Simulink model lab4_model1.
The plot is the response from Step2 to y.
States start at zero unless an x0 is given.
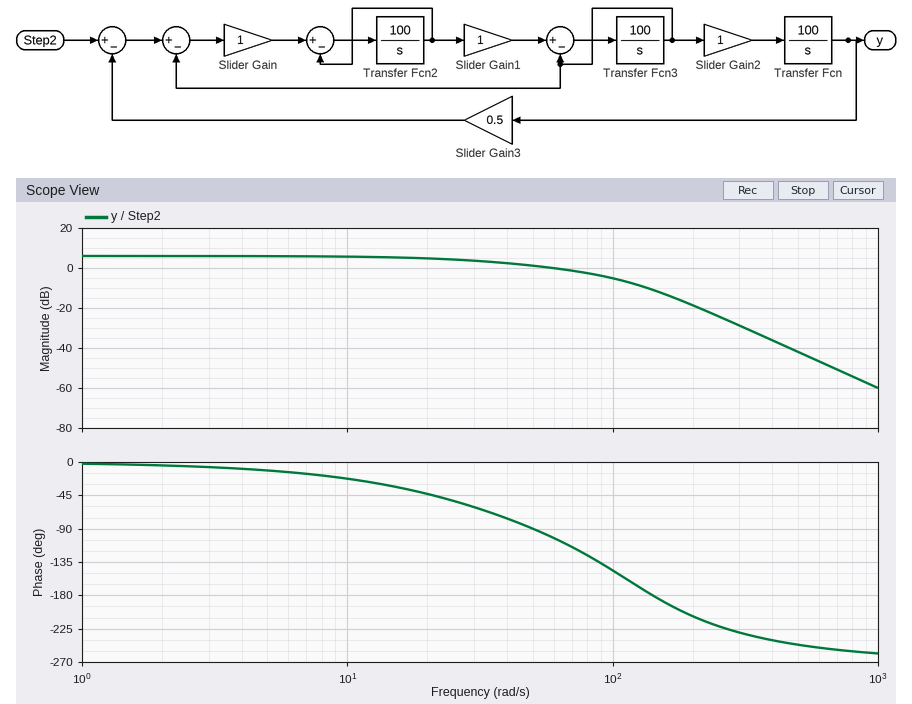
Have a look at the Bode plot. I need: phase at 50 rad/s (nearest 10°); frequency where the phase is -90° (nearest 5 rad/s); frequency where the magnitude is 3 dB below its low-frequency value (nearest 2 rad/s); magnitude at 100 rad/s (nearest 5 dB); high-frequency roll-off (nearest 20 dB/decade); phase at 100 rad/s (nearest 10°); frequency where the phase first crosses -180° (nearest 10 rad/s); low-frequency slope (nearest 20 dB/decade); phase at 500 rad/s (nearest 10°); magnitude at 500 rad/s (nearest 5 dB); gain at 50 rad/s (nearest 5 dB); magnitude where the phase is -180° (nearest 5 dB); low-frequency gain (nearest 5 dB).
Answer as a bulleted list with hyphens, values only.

- -90°
- 50 rad/s
- 36 rad/s
- -5 dB
- -60 dB/decade
- -150°
- 140 rad/s
- 0 dB/decade
- -250°
- -40 dB
- 0 dB
- -10 dB
- 5 dB
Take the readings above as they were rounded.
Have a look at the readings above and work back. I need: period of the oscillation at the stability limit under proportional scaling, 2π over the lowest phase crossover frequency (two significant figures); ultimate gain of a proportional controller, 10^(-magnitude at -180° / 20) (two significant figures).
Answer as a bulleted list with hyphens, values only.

- 0.045 s
- 3.2
